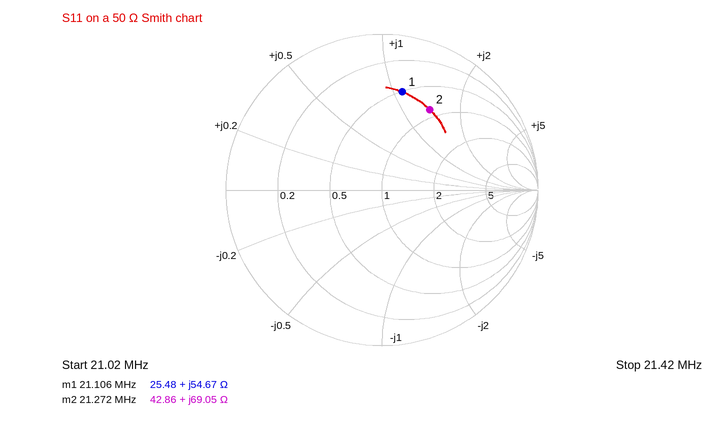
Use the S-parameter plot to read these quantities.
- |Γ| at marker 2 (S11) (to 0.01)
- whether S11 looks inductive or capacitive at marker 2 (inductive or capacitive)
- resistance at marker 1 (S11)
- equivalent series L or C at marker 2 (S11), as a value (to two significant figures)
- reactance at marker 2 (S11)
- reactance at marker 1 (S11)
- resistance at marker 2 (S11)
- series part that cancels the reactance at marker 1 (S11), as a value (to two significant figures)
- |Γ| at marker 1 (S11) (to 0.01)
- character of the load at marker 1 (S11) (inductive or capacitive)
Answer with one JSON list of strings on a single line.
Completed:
["0.60", "inductive", "25.48 Ω", "520 nH", "+69.05 Ω", "+54.67 Ω", "42.86 Ω", "140 pF", "0.64", "inductive"]
